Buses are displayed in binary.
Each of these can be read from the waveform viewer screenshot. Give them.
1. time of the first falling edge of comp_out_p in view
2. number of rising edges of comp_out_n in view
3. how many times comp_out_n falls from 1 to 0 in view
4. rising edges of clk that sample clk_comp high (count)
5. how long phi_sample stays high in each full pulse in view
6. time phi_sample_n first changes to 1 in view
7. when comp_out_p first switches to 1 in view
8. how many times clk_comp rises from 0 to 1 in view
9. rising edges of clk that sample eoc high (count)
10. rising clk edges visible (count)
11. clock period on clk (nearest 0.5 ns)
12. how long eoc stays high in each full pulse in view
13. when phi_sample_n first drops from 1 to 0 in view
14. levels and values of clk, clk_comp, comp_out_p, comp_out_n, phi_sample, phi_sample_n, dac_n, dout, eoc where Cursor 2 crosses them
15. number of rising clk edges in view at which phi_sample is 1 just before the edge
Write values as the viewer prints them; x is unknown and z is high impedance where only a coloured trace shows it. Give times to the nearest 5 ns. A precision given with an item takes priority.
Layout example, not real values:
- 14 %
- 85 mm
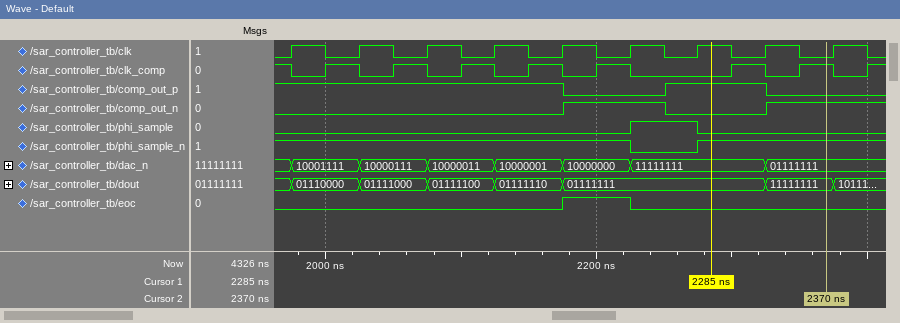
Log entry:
- 2175 ns
- 2
- 1
- 8
- 50 ns
- 2275 ns
- 2250 ns
- 8
- 1
- 9
- 50 ns
- 50 ns
- 2225 ns
- clk=0, clk_comp=1, comp_out_p=0, comp_out_n=1, phi_sample=0, phi_sample_n=1, dac_n=01111111, dout=11111111, eoc=0
- 1
